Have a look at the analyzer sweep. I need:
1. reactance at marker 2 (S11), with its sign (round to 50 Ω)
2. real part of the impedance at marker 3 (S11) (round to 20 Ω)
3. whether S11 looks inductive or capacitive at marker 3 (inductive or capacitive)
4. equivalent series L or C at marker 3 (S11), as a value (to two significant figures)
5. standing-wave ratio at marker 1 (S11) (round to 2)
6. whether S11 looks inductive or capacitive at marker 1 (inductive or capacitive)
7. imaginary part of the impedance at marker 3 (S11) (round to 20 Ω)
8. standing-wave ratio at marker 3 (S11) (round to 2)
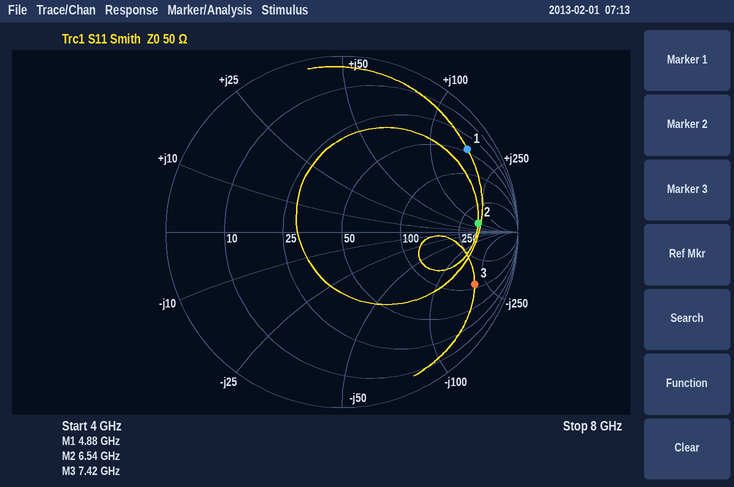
+100 Ω
120 Ω
capacitive
110 fF
12
inductive
-200 Ω
10
